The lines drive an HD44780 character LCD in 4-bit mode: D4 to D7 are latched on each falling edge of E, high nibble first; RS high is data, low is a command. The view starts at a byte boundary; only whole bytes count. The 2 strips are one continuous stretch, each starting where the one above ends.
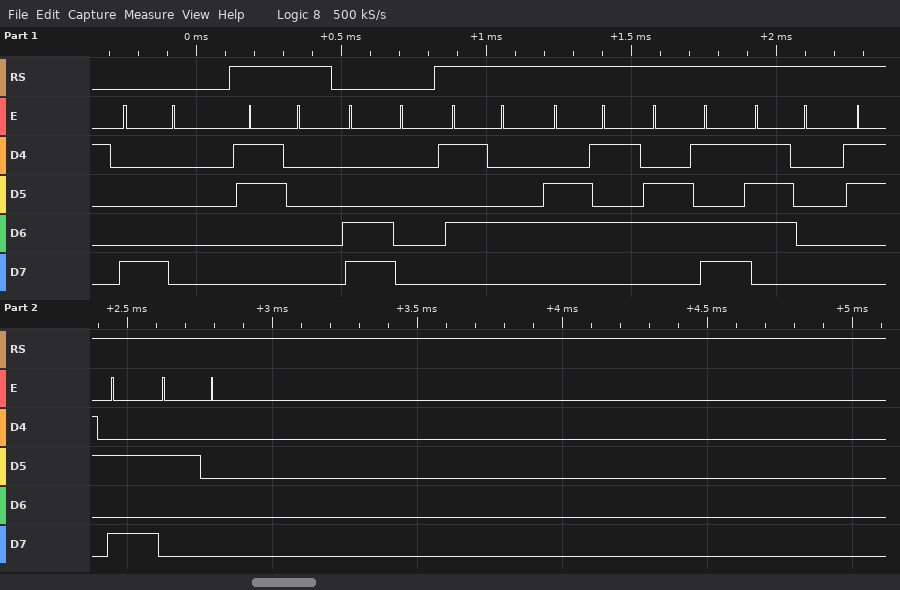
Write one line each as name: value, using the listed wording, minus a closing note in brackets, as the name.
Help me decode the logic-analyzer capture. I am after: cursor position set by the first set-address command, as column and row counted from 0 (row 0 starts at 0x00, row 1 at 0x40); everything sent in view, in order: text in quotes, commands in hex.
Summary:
cursor position set by the first set-address command, as column and row counted from 0: column 0, row 0
everything sent in view, in order: text in quotes, commands in hex: 0x80 "0" 0xC0 "Temp: "
